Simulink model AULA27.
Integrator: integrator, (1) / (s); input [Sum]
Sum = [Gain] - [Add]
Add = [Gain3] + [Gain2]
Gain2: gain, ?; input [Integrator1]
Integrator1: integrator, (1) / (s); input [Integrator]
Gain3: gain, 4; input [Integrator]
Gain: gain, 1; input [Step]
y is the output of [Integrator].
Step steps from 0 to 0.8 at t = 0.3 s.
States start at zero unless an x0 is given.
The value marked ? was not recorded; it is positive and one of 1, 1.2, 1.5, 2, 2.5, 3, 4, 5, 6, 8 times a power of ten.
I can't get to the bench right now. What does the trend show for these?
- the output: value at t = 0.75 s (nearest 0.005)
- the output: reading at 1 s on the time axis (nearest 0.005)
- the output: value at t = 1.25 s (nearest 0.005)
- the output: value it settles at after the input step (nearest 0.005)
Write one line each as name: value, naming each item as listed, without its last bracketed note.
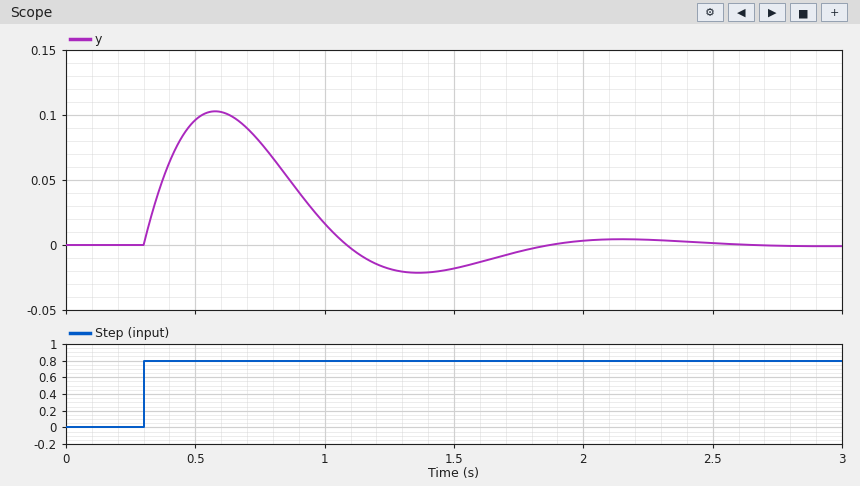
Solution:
the output: value at t = 0.75 s: 0.080
the output: reading at 1 s on the time axis: 0.015
the output: value at t = 1.25 s: -0.020
the output: value it settles at after the input step: 0.000
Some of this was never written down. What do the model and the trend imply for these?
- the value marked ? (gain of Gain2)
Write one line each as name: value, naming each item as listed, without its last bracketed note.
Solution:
the value marked ?: 20
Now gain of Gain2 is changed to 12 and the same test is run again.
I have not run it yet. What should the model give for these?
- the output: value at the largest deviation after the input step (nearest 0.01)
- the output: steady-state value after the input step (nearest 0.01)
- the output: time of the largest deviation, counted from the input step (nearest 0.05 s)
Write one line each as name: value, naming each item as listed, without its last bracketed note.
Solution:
the output: value at the largest deviation after the input step: 0.12
the output: steady-state value after the input step: 0.00
the output: time of the largest deviation, counted from the input step: 0.35 s
